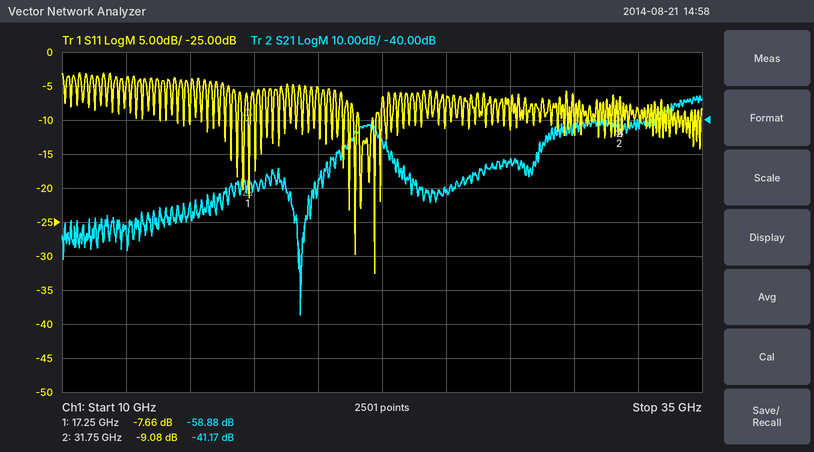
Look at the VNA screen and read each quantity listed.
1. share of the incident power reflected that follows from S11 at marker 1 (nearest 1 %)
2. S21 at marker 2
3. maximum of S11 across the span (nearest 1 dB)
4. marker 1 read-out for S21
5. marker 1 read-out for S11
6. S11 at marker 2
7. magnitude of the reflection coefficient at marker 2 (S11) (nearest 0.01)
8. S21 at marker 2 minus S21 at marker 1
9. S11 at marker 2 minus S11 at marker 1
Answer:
17 %
-41.17 dB
-3 dB
-58.88 dB
-7.66 dB
-9.08 dB
0.35
17.71 dB
-1.42 dB
